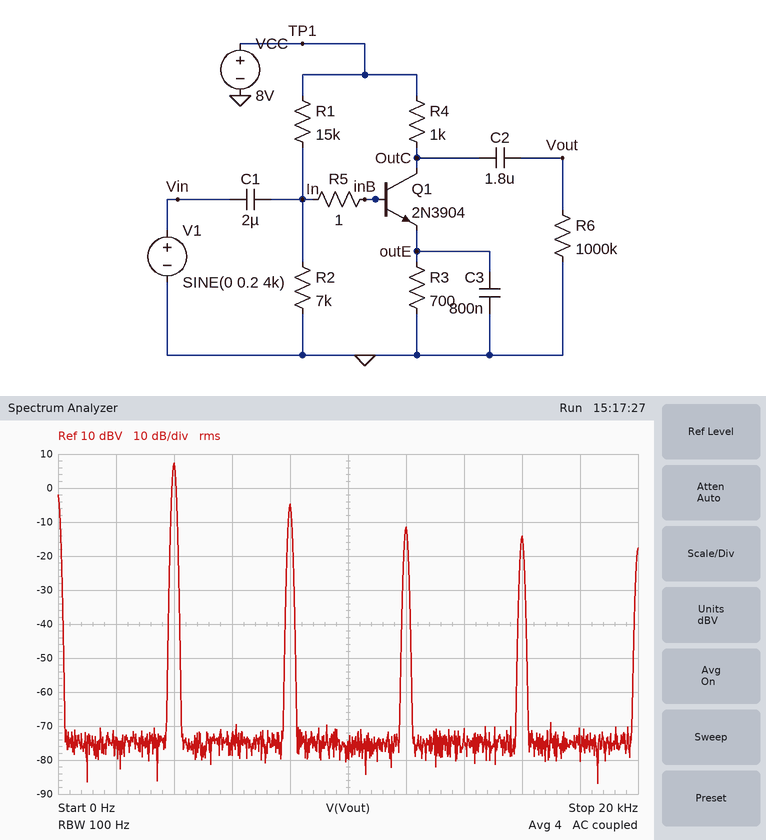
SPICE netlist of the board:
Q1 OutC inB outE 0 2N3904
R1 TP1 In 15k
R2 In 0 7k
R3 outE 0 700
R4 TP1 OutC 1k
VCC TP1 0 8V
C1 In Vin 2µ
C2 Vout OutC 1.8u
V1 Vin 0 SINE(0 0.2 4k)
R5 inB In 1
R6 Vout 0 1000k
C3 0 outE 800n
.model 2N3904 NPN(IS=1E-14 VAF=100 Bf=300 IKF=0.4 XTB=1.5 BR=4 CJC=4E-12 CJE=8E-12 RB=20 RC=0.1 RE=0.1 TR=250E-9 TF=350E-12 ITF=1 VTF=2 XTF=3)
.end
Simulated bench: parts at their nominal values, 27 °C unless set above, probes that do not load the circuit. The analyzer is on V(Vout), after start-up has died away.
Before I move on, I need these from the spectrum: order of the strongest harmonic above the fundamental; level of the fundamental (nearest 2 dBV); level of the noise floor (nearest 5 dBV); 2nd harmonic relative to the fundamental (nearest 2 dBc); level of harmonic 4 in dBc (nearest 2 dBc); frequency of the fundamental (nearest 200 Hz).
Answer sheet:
2
8 dBV
-75 dBV
-12 dBc
-22 dBc
4.0 kHz
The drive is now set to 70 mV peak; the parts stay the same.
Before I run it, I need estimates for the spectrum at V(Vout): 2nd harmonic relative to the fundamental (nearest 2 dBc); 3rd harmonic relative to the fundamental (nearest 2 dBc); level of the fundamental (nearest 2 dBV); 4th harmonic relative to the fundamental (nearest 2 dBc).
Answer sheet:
-26 dBc
-38 dBc
0 dBV
-52 dBc
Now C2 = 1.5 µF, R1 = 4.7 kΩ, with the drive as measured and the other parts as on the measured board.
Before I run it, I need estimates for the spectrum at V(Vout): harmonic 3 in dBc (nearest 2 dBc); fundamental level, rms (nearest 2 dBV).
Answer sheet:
-18 dBc
6 dBV
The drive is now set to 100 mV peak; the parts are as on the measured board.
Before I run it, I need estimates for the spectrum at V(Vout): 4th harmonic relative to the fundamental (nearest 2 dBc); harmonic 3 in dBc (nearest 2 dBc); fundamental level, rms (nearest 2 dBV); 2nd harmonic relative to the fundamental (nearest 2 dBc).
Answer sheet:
-42 dBc
-32 dBc
2 dBV
-22 dBc
